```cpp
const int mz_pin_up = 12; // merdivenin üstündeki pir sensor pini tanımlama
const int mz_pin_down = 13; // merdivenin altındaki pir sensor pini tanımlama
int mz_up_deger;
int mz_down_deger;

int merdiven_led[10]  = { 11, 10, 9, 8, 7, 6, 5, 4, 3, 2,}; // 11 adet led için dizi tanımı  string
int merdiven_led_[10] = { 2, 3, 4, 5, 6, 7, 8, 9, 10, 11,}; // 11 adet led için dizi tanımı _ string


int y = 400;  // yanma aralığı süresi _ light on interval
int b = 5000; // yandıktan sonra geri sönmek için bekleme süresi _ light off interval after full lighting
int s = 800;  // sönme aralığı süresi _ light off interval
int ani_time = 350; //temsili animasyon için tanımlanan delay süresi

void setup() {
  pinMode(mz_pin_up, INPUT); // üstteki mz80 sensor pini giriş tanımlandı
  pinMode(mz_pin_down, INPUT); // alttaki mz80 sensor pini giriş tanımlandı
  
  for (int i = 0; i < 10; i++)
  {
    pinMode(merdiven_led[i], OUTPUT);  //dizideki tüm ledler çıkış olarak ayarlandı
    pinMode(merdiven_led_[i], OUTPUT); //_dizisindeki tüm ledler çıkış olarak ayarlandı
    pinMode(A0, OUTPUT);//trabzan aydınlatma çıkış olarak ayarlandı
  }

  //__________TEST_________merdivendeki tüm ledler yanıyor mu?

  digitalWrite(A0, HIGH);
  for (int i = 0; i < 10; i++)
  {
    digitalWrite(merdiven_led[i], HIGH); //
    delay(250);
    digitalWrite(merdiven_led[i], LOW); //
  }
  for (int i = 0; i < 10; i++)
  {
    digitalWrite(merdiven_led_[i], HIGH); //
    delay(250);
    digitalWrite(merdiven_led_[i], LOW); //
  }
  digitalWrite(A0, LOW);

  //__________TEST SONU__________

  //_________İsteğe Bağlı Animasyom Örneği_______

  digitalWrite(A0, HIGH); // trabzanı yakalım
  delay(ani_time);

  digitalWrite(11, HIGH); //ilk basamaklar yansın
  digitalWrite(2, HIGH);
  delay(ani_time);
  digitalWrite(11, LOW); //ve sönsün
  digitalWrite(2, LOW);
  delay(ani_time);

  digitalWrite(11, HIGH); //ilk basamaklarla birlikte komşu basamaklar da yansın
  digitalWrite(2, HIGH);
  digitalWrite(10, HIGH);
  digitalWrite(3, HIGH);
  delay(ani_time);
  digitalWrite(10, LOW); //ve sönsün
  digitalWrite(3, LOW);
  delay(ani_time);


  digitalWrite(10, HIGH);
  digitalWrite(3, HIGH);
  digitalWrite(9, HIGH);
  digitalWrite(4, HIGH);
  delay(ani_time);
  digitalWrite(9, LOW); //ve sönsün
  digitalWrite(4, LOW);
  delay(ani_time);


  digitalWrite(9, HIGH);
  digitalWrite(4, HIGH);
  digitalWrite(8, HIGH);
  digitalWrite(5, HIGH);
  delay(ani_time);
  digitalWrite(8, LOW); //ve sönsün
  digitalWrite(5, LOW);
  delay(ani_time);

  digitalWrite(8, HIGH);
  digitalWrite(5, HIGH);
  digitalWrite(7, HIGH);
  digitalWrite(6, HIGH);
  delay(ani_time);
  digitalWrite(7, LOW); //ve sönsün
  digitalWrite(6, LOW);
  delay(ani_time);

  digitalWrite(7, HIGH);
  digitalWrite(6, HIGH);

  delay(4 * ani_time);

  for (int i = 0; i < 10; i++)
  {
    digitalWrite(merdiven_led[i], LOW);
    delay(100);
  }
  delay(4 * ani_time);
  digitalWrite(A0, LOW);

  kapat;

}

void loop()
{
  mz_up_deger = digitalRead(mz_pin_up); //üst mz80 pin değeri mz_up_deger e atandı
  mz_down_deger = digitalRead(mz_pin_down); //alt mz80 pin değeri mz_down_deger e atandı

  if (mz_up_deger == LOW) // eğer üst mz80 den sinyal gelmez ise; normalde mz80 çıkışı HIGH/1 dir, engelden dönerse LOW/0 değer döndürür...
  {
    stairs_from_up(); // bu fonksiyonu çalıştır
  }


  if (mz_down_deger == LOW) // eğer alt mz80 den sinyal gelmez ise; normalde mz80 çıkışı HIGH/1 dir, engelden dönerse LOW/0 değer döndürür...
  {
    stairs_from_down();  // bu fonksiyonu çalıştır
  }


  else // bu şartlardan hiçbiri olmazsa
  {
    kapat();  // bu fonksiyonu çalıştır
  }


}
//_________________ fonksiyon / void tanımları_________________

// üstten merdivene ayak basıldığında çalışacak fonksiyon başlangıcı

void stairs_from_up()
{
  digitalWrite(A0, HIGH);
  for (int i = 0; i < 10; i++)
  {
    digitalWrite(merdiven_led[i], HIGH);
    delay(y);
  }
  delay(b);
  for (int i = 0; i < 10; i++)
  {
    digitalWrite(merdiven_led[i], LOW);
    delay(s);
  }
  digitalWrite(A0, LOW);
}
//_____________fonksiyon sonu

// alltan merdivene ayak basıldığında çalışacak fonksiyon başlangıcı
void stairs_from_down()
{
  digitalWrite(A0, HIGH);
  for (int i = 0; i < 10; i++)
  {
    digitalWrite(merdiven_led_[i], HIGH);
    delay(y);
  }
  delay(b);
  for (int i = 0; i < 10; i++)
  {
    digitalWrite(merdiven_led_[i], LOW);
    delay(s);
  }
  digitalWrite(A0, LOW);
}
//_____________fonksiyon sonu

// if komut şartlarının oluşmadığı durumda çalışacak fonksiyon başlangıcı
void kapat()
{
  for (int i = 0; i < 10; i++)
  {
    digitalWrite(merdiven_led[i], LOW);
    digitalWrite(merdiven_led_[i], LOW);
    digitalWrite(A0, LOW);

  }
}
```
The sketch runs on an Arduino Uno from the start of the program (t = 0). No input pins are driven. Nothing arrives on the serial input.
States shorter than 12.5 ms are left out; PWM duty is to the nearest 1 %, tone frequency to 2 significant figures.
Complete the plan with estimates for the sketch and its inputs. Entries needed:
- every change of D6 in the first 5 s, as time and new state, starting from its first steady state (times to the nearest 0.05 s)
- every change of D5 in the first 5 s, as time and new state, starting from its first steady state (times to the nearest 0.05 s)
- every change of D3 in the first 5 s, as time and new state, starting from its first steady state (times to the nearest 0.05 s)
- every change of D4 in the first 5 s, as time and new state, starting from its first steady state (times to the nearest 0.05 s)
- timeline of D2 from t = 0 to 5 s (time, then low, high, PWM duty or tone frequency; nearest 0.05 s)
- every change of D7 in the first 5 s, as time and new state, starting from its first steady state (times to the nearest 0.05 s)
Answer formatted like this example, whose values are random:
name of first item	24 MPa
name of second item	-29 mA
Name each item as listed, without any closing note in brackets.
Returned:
every change of D6 in the first 5 s, as time and new state, starting from its first steady state	0 s low; 1.25 s high; 1.5 s low; 3.5 s high; 3.75 s low
every change of D5 in the first 5 s, as time and new state, starting from its first steady state	0 s low; 1.5 s high; 1.75 s low; 3.25 s high; 3.5 s low
every change of D3 in the first 5 s, as time and new state, starting from its first steady state	0 s low; 2 s high; 2.25 s low; 2.75 s high; 3 s low
every change of D4 in the first 5 s, as time and new state, starting from its first steady state	0 s low; 1.75 s high; 2 s low; 3 s high; 3.25 s low
timeline of D2 from t = 0 to 5 s	0 s low; 2.25 s high; 2.75 s low
every change of D7 in the first 5 s, as time and new state, starting from its first steady state	0 s low; 1 s high; 1.25 s low; 3.75 s high; 4 s low
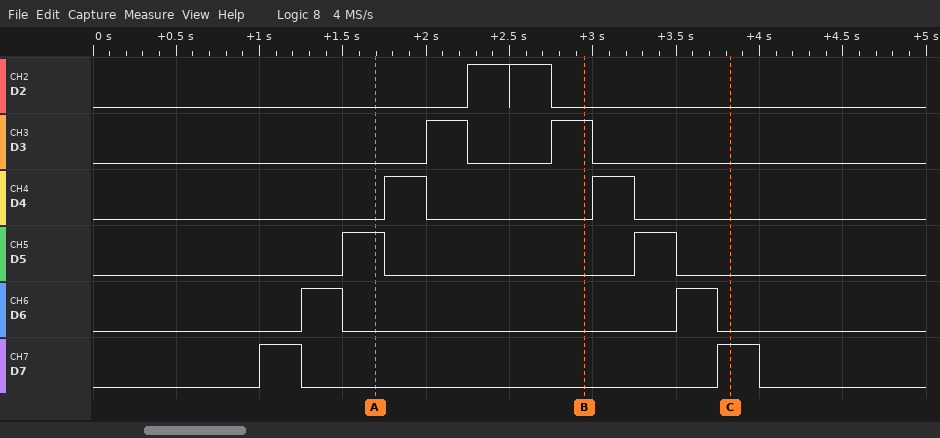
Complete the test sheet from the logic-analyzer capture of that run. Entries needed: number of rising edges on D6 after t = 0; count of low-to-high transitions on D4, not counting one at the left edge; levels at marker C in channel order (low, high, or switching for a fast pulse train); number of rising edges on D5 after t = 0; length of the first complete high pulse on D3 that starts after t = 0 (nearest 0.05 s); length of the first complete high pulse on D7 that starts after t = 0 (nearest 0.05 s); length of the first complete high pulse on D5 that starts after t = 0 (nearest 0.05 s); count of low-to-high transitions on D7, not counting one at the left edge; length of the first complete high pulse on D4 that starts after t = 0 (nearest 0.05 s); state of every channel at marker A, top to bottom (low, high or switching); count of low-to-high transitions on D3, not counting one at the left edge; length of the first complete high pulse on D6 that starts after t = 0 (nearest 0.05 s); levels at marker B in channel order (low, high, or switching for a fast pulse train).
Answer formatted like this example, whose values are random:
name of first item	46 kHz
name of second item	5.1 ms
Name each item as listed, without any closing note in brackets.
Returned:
number of rising edges on D6 after t = 0	2
count of low-to-high transitions on D4, not counting one at the left edge	2
levels at marker C in channel order	D2 low, D3 low, D4 low, D5 low, D6 low, D7 high
number of rising edges on D5 after t = 0	2
length of the first complete high pulse on D3 that starts after t = 0	0.25 s
length of the first complete high pulse on D7 that starts after t = 0	0.25 s
length of the first complete high pulse on D5 that starts after t = 0	0.25 s
count of low-to-high transitions on D7, not counting one at the left edge	2
length of the first complete high pulse on D4 that starts after t = 0	0.25 s
state of every channel at marker A, top to bottom	D2 low, D3 low, D4 low, D5 high, D6 low, D7 low
count of low-to-high transitions on D3, not counting one at the left edge	2
length of the first complete high pulse on D6 that starts after t = 0	0.25 s
levels at marker B in channel order	D2 low, D3 high, D4 low, D5 low, D6 low, D7 low
